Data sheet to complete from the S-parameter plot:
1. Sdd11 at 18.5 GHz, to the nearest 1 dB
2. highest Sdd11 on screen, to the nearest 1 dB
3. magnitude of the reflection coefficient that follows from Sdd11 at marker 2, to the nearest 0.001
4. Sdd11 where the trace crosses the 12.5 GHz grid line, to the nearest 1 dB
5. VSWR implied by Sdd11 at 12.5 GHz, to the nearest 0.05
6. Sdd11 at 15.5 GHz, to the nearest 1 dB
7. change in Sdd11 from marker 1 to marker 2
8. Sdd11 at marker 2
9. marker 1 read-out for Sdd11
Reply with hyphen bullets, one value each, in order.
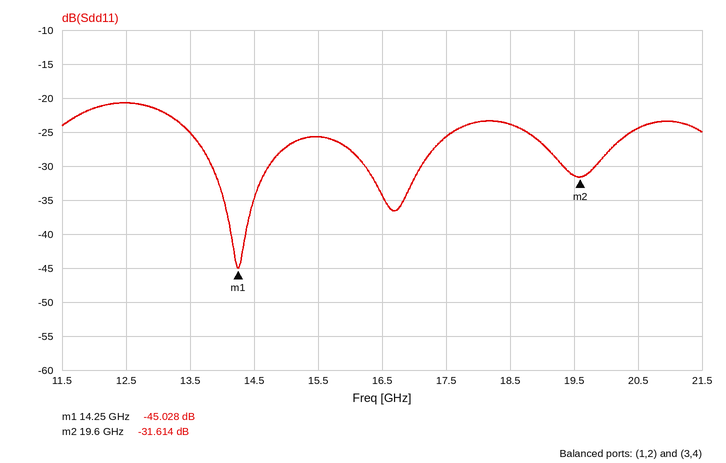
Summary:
- -24 dB
- -21 dB
- 0.026
- -21 dB
- 1.20
- -26 dB
- 13.414 dB
- -31.614 dB
- -45.028 dB
